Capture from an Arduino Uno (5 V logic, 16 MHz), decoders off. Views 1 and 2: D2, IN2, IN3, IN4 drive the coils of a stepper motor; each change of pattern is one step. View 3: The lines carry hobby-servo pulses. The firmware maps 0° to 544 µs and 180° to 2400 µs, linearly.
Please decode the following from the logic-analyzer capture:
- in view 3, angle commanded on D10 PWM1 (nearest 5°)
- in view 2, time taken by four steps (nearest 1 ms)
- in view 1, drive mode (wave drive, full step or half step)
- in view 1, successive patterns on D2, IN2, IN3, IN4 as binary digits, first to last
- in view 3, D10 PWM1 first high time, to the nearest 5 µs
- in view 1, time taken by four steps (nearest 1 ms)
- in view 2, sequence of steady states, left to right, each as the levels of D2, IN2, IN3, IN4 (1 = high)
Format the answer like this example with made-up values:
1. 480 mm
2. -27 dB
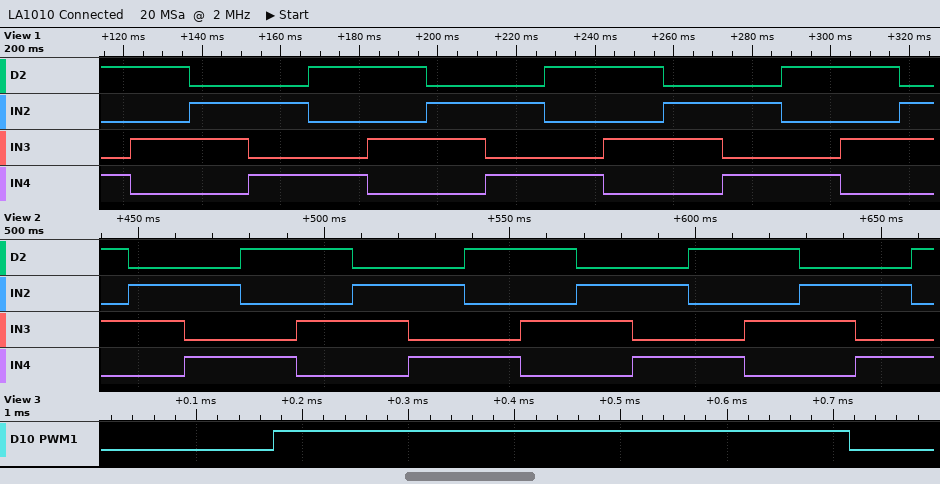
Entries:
1. 0°
2. 60 ms
3. full step
4. 1001 1010 0110 0101 1001 1010 0110 0101 1001 1010 0110 0101 1001 1010 0110
5. 545 µs
6. 60 ms
7. 1010 0110 0101 1001 1010 0110 0101 1001 1010 0110 0101 1001 1010 0110 0101 1001
